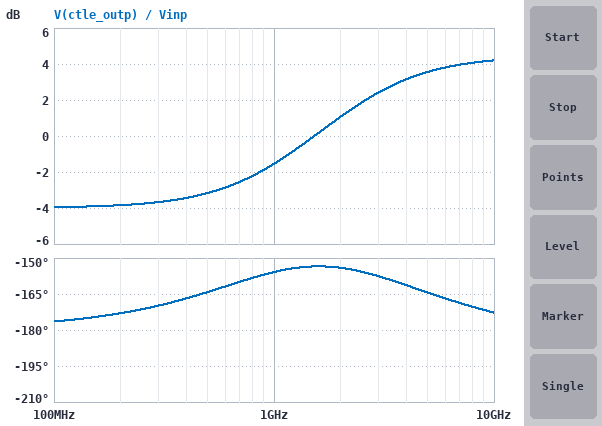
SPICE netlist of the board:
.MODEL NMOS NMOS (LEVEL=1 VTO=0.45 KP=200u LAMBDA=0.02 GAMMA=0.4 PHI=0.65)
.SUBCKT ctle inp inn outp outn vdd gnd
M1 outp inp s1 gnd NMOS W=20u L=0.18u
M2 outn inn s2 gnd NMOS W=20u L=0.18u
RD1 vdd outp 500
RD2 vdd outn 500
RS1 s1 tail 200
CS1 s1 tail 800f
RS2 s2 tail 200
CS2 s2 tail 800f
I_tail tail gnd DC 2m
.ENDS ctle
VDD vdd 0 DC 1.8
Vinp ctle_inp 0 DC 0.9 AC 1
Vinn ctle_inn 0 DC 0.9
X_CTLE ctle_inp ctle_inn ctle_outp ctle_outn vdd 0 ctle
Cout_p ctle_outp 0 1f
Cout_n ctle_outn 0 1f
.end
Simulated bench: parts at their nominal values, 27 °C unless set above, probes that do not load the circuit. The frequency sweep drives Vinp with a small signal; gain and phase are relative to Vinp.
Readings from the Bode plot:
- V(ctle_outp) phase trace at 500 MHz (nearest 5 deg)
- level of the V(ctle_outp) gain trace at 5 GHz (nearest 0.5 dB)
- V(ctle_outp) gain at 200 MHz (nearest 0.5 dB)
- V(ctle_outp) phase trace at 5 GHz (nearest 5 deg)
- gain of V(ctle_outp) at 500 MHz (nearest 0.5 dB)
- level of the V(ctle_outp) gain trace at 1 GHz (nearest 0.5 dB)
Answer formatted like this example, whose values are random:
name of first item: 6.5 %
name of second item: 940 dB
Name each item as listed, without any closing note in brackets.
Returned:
V(ctle_outp) phase trace at 500 MHz: -165 deg
level of the V(ctle_outp) gain trace at 5 GHz: 3.5 dB
V(ctle_outp) gain at 200 MHz: -4.0 dB
V(ctle_outp) phase trace at 5 GHz: -165 deg
gain of V(ctle_outp) at 500 MHz: -3.0 dB
level of the V(ctle_outp) gain trace at 1 GHz: -1.5 dB
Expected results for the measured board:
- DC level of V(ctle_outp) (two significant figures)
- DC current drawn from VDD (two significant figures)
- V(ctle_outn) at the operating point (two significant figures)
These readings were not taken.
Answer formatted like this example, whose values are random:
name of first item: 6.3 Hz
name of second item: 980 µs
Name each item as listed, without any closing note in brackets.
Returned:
DC level of V(ctle_outp): 1.3 V
DC current drawn from VDD: 2.0 mA
V(ctle_outn) at the operating point: 1.3 V
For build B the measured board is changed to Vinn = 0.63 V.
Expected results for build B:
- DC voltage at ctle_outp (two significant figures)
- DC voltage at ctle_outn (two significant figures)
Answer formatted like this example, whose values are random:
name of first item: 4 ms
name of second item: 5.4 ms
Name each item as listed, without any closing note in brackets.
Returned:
DC voltage at ctle_outp: 1.1 V
DC voltage at ctle_outn: 1.5 V
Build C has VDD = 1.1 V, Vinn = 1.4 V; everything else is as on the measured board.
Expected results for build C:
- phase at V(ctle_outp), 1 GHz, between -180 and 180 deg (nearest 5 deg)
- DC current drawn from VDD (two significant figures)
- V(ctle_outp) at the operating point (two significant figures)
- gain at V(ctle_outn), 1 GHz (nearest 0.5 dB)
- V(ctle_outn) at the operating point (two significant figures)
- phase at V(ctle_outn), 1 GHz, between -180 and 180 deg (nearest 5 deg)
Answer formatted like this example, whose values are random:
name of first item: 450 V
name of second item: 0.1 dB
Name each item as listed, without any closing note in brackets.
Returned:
phase at V(ctle_outp), 1 GHz, between -180 and 180 deg: -165 deg
DC current drawn from VDD: 2.0 mA
V(ctle_outp) at the operating point: 770 mV
gain at V(ctle_outn), 1 GHz: -6.0 dB
V(ctle_outn) at the operating point: 430 mV
phase at V(ctle_outn), 1 GHz, between -180 and 180 deg: 15 deg
